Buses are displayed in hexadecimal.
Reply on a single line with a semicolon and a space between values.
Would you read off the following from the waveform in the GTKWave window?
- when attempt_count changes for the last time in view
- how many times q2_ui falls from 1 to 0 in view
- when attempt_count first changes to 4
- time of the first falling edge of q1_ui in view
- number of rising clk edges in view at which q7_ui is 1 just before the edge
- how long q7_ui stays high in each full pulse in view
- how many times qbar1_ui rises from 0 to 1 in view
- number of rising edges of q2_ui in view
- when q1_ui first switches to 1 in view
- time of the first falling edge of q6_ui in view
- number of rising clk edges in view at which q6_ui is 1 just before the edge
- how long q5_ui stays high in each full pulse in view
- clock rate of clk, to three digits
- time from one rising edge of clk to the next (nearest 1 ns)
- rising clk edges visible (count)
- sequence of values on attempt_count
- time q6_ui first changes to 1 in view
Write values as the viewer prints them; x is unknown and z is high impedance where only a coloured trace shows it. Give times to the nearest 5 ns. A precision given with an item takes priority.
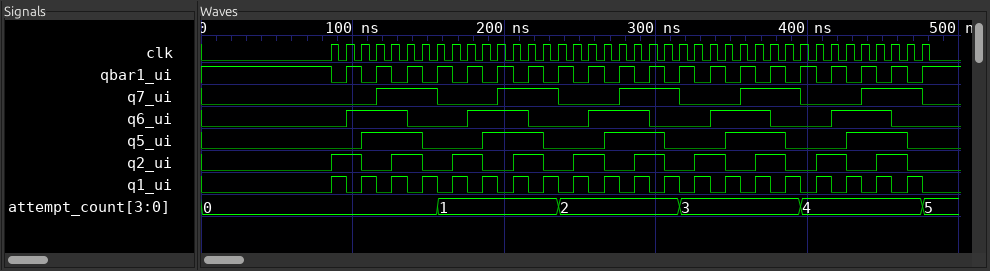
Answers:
475 ns; 10; 395 ns; 95 ns; 20; 40 ns, 40 ns, 40 ns, 40 ns, 40 ns; 20; 10; 85 ns; 135 ns; 20; 40 ns, 40 ns, 40 ns, 40 ns, 40 ns; 100 MHz; 10 ns; 40; 0, 1, 2, 3, 4, 5; 95 ns
